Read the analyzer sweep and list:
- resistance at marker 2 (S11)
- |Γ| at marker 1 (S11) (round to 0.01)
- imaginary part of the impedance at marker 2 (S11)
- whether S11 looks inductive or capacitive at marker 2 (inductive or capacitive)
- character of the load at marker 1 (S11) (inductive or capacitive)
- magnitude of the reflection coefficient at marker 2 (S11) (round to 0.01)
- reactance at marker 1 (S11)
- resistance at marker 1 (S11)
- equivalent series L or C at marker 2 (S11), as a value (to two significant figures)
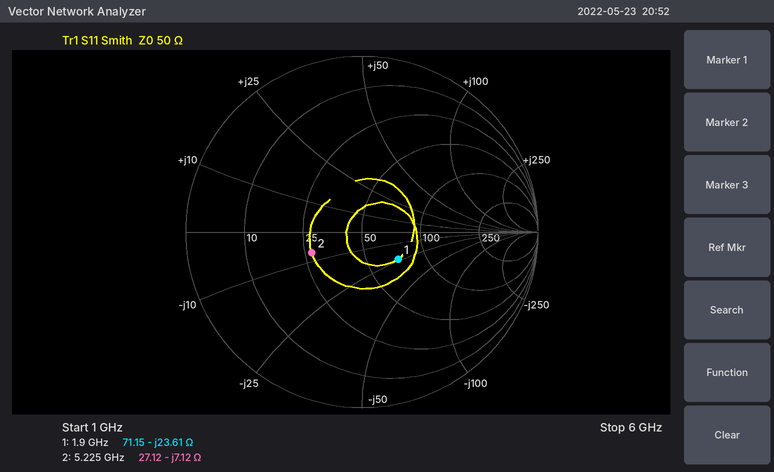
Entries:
27.12 Ω
0.26
-7.12 Ω
capacitive
capacitive
0.31
-23.61 Ω
71.15 Ω
4.3 pF
